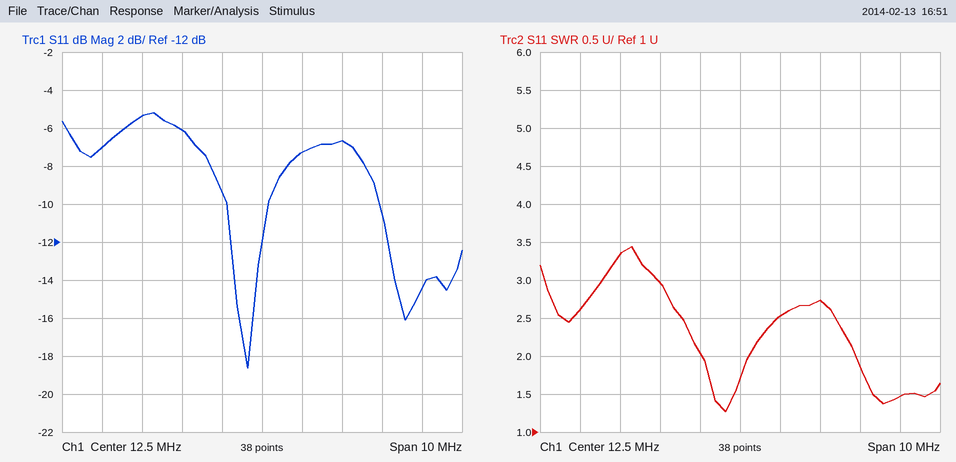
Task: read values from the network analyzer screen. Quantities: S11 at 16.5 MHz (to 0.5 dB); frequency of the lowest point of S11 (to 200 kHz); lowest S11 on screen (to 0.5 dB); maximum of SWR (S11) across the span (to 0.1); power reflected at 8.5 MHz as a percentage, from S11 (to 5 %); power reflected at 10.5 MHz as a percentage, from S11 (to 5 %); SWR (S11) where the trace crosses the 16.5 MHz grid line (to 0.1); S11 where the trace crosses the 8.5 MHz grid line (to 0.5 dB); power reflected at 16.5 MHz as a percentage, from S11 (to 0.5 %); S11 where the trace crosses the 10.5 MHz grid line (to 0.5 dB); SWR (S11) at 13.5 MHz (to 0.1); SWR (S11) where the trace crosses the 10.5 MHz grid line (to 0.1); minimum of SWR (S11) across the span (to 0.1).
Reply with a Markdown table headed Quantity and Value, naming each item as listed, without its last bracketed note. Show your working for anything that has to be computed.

| Quantity | Value |
|---|---|
| S11 at 16.5 MHz | -14.5 dB |
| frequency of the lowest point of S11 | 12.2 MHz |
| lowest S11 on screen | -18.5 dB |
| maximum of SWR (S11) across the span | 3.4 |
| power reflected at 8.5 MHz as a percentage, from S11 | 10^(-7/10) ≈ 20 % |
| power reflected at 10.5 MHz as a percentage, from S11 | 10^(-6/10) ≈ 25 % |
| SWR (S11) where the trace crosses the 16.5 MHz grid line | 1.5 |
| S11 where the trace crosses the 8.5 MHz grid line | -7.0 dB |
| power reflected at 16.5 MHz as a percentage, from S11 | 10^(-14.5/10) ≈ 3.5 % |
| S11 where the trace crosses the 10.5 MHz grid line | -6.0 dB |
| SWR (S11) at 13.5 MHz | 2.5 |
| SWR (S11) where the trace crosses the 10.5 MHz grid line | 3.0 |
| minimum of SWR (S11) across the span | 1.3 |
